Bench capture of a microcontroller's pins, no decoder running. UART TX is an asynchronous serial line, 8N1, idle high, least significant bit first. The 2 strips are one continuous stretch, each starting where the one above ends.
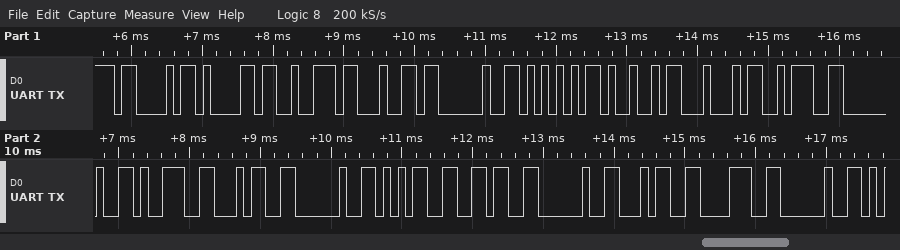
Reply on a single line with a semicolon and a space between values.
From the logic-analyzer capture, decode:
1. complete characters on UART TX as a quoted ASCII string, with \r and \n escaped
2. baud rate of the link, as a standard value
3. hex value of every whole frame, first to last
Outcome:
"Card UID: 94 56 48 "; 9600 baud; 43 61 72 64 20 55 49 44 3A 20 39 34 20 35 36 20 34 38 20
